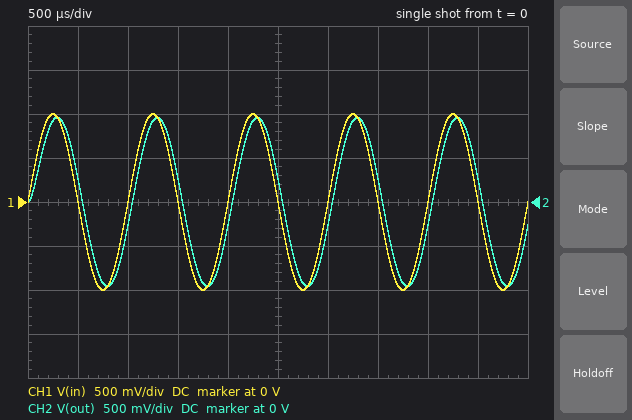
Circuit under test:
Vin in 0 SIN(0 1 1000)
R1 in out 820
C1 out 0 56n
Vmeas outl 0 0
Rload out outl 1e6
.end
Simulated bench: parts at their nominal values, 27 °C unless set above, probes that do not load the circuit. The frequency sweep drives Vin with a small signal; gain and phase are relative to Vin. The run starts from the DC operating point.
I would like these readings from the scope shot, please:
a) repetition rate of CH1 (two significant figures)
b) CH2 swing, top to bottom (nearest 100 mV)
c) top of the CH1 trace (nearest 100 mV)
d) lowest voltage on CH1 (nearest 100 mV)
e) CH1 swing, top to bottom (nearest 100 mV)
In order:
1.0 kHz
1.9 V
1.0 V
-1.0 V
2.0 V
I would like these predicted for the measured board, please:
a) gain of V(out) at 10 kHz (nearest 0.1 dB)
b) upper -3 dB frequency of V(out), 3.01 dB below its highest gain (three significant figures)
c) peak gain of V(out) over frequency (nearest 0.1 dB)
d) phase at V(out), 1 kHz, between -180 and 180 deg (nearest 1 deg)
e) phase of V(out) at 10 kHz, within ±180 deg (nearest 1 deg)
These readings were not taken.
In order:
-9.7 dB
3.47 kHz
0 dB
-16 deg
-71 deg
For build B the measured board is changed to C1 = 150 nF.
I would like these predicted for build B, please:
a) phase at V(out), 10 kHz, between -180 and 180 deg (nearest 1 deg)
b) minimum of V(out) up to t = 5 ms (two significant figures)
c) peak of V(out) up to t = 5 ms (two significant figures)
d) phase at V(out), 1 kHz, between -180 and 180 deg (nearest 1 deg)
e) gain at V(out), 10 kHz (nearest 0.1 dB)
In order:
-83 deg
-790 mV
820 mV
-38 deg
-17.8 dB
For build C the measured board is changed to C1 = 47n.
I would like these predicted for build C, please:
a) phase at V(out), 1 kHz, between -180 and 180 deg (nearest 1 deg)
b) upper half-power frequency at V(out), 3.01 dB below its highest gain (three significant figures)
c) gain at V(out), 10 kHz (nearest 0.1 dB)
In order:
-14 deg
4.13 kHz
-8.4 dB
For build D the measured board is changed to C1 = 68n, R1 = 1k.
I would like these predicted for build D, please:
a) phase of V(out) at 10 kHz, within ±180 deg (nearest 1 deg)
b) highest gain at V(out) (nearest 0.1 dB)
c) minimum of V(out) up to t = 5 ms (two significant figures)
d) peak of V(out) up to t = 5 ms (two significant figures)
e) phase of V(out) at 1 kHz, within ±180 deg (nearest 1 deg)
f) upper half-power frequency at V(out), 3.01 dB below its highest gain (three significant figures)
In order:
-77 deg
0 dB
-920 mV
920 mV
-23 deg
2.34 kHz
